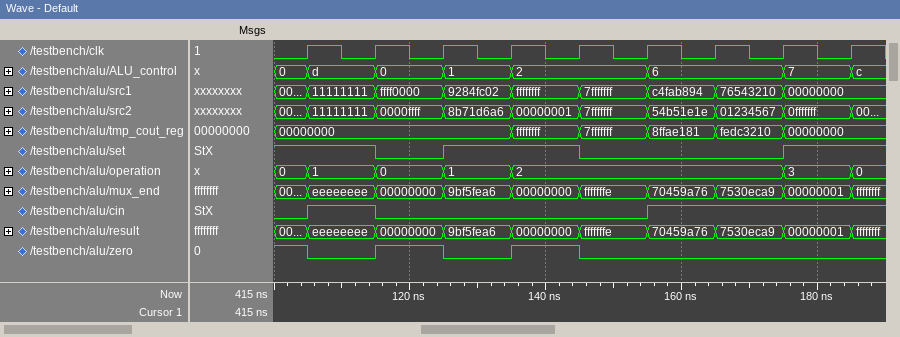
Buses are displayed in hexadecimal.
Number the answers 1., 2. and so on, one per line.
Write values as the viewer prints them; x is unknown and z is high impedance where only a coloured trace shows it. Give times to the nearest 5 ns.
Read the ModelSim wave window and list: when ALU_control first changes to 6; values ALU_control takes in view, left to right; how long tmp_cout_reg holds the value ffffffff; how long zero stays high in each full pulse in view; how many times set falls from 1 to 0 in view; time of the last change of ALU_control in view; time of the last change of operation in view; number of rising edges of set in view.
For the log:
1. 155 ns
2. 0, d, 0, 1, 2, 6, 7, c
3. 10 ns
4. 10 ns, 10 ns
5. 2
6. 185 ns
7. 185 ns
8. 2
